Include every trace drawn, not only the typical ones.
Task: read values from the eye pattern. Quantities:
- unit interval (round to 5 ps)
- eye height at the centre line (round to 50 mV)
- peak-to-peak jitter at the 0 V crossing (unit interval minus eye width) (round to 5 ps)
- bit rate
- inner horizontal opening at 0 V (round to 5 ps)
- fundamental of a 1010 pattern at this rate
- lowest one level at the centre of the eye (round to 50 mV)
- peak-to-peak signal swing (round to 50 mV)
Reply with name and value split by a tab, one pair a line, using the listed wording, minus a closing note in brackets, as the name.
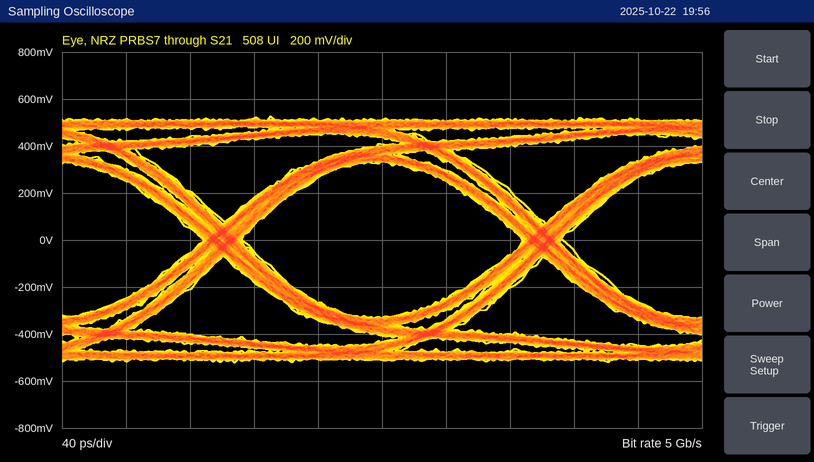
unit interval	200 ps
eye height at the centre line	650 mV
peak-to-peak jitter at the 0 V crossing (unit interval minus eye width)	25 ps
bit rate	5 Gb/s
inner horizontal opening at 0 V	175 ps
fundamental of a 1010 pattern at this rate	2.5 GHz
lowest one level at the centre of the eye	350 mV
peak-to-peak signal swing	1.05 V
